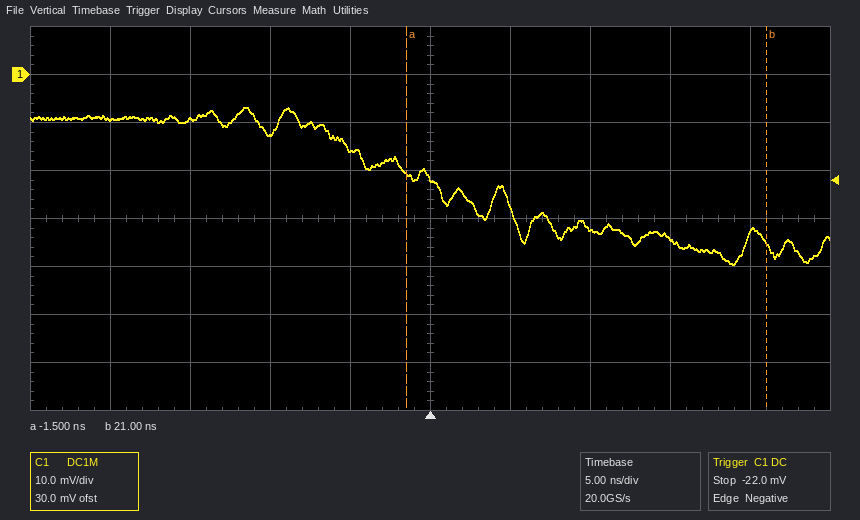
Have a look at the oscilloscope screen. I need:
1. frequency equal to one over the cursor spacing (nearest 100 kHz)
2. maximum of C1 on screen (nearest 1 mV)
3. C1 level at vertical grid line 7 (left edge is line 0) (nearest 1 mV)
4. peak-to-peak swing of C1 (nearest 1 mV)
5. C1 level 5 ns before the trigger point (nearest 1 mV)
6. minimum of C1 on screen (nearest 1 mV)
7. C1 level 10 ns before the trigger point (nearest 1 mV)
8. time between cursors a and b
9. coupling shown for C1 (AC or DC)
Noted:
44.4 MHz
-7 mV
-32 mV
33 mV
-15 mV
-40 mV
-12 mV
22.5 ns
DC
